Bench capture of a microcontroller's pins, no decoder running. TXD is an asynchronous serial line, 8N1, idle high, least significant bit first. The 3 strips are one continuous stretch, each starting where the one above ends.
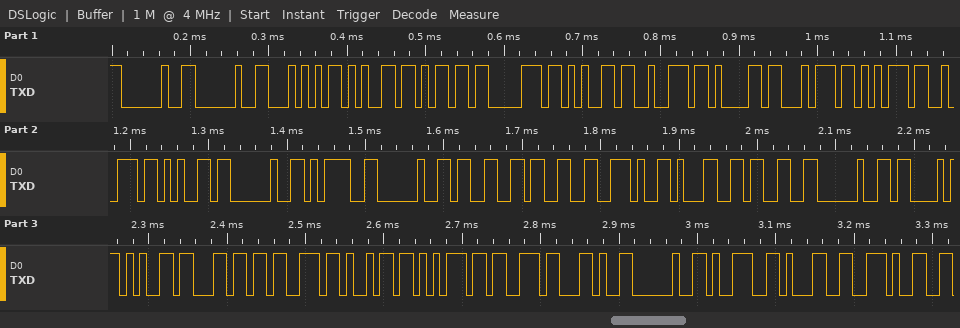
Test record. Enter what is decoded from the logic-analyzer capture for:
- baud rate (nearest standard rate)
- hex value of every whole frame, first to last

115200 baud
0x20 0x20 0x54 0x65 0x6D 0x70 0x65 0x72 0x61 0x74 0x75 0x72 0x65 0x20 0x3D 0x20 0x33 0x33 0x2E 0x31 0x33 0x20 0x43 0x65 0x6C 0x73 0x69 0x75 0x73 0x2C 0x20 0x39 0x31 0x2E
